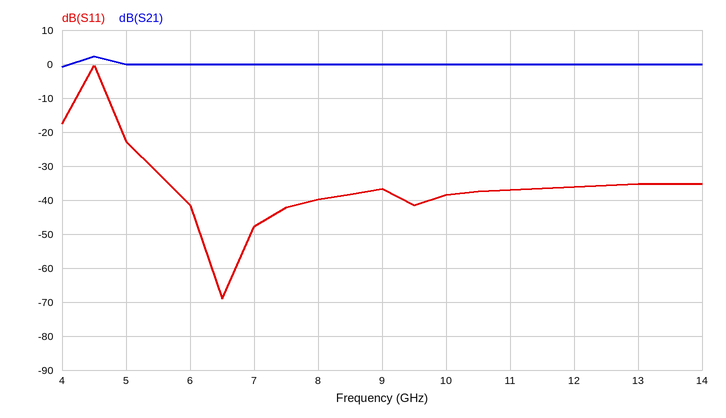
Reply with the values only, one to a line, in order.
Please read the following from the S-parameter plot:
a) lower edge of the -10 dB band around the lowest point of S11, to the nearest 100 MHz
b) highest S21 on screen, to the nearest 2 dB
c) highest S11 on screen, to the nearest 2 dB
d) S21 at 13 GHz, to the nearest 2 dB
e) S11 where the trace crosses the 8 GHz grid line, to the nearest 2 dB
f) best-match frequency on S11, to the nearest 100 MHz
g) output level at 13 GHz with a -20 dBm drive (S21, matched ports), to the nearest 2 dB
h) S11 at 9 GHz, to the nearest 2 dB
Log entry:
4.7 GHz
2 dB
0 dB
0 dB
-40 dB
6.5 GHz
-20 dBm
-36 dB
